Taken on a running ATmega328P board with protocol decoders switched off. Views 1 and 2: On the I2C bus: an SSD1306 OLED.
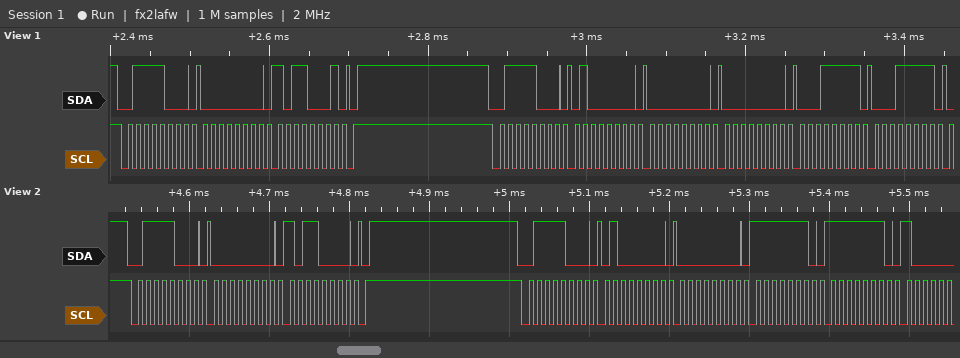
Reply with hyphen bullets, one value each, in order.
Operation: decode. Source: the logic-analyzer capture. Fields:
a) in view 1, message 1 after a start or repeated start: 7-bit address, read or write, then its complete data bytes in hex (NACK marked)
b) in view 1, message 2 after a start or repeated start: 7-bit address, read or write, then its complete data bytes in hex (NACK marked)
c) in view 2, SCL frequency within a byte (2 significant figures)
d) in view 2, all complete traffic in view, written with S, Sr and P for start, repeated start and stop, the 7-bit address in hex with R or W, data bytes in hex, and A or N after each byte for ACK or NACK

- 0x3C write: 00 B1
- 0x3C write: 40 00 00 1F 1F
- 100 kHz
- S 3CW A 00 A B0 A P S 3CW A 40 A 00 A FE A FE A
